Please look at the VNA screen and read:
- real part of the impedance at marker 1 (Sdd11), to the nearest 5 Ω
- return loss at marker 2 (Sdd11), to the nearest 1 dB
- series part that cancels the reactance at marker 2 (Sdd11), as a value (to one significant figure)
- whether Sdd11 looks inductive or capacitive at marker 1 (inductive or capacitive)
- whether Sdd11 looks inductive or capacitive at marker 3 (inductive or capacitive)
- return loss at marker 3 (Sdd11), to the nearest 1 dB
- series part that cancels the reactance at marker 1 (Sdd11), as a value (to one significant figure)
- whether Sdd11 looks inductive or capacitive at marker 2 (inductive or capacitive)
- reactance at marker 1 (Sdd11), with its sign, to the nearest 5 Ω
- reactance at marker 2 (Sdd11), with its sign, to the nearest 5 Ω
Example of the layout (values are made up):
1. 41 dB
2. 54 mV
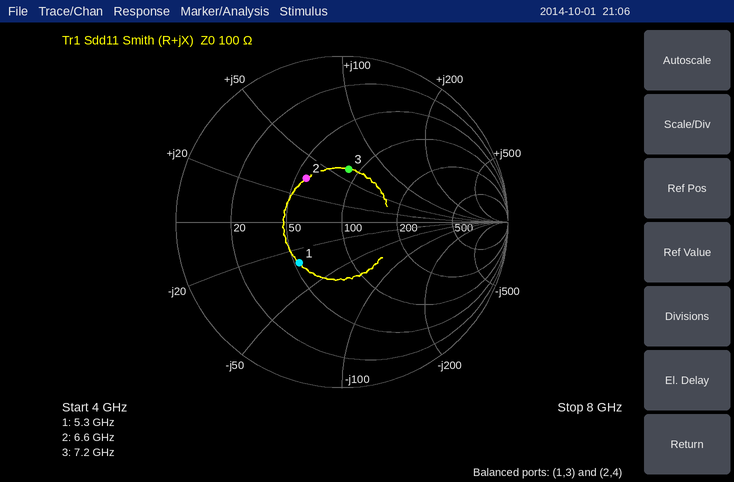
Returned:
1. 55 Ω
2. 9 dB
3. 700 fF
4. capacitive
5. inductive
6. 10 dB
7. 900 pH
8. inductive
9. -30 Ω
10. +35 Ω
